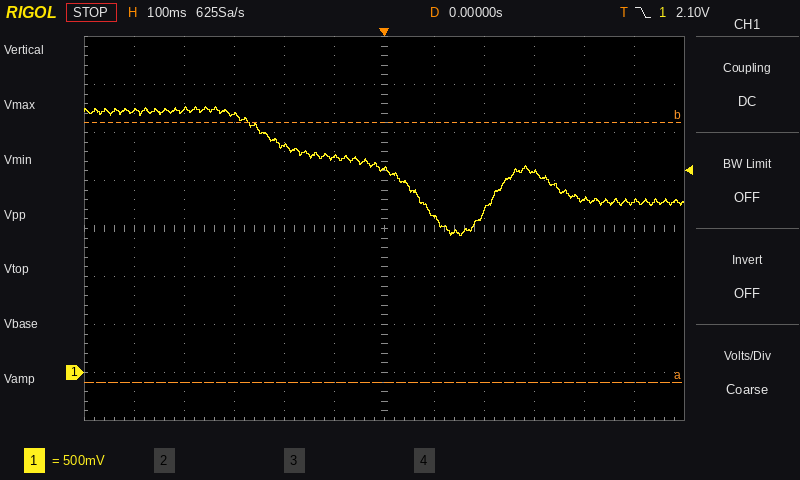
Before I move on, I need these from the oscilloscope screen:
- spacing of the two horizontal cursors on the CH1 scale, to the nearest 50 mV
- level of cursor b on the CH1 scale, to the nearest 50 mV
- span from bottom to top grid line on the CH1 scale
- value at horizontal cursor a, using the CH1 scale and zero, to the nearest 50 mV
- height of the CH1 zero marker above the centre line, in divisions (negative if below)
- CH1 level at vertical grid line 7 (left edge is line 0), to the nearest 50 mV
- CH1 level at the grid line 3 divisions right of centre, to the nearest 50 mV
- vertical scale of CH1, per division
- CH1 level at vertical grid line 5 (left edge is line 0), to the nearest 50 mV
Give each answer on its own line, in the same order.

2.70 V
2.60 V
4 V
-100 mV
-3.0 div
1.60 V
2.10 V
500 mV
2.25 V
